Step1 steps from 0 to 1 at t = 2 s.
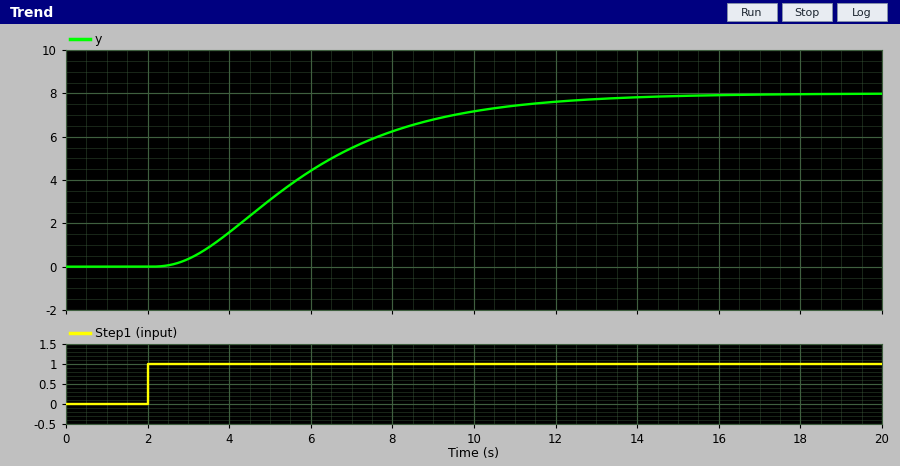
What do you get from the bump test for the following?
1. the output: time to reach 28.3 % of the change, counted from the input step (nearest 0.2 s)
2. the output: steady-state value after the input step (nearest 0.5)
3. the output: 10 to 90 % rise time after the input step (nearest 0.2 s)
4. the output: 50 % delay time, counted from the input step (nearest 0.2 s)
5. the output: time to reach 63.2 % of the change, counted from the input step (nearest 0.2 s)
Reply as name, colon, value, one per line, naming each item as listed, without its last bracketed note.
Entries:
the output: time to reach 28.3 % of the change, counted from the input step: 2.4 s
the output: steady-state value after the input step: 8.0
the output: 10 to 90 % rise time after the input step: 6.6 s
the output: 50 % delay time, counted from the input step: 3.6 s
the output: time to reach 63.2 % of the change, counted from the input step: 4.6 s
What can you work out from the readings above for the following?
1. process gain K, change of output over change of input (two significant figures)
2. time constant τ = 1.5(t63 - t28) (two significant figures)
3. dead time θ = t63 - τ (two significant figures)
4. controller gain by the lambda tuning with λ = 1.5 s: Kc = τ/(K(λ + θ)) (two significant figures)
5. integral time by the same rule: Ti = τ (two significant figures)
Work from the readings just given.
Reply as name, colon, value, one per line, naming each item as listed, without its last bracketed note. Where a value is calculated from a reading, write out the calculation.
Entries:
process gain K, change of output over change of input: (8 - 0) / 1 = 8.0
time constant τ = 1.5(t63 - t28): 1.5 × (4.6 - 2.4) = 3.3 s
dead time θ = t63 - τ: 4.6 - 3.3 = 1.3 s
controller gain by the lambda tuning with λ = 1.5 s: Kc = τ/(K(λ + θ)): 3.3 / (8 × (1.5 + 1.3)) = 0.15
integral time by the same rule: Ti = τ: 3.3 s
